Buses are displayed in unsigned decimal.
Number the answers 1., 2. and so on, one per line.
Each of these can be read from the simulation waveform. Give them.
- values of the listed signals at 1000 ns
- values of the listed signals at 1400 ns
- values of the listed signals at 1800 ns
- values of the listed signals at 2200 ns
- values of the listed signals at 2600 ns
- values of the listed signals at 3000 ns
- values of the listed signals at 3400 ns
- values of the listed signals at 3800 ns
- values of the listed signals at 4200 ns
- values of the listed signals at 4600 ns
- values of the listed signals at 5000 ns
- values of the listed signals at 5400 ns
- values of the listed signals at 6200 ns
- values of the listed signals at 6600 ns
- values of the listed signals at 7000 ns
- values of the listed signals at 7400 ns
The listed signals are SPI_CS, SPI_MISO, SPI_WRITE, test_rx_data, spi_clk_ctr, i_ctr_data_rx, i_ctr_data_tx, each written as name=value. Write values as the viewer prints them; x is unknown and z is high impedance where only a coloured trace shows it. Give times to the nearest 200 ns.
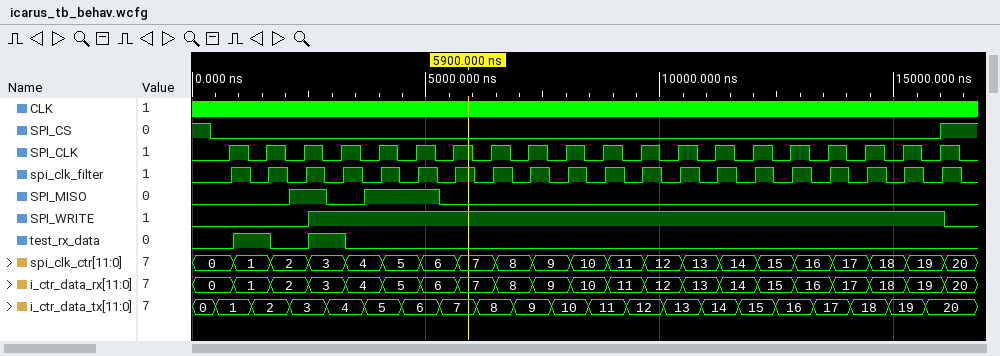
1. SPI_CS=0, SPI_MISO=0, SPI_WRITE=0, test_rx_data=1, spi_clk_ctr=1, i_ctr_data_rx=1, i_ctr_data_tx=1
2. SPI_CS=0, SPI_MISO=0, SPI_WRITE=0, test_rx_data=1, spi_clk_ctr=1, i_ctr_data_rx=1, i_ctr_data_tx=2
3. SPI_CS=0, SPI_MISO=0, SPI_WRITE=0, test_rx_data=0, spi_clk_ctr=2, i_ctr_data_rx=2, i_ctr_data_tx=2
4. SPI_CS=0, SPI_MISO=1, SPI_WRITE=0, test_rx_data=0, spi_clk_ctr=2, i_ctr_data_rx=2, i_ctr_data_tx=3
5. SPI_CS=0, SPI_MISO=1, SPI_WRITE=1, test_rx_data=1, spi_clk_ctr=3, i_ctr_data_rx=3, i_ctr_data_tx=3
6. SPI_CS=0, SPI_MISO=0, SPI_WRITE=1, test_rx_data=1, spi_clk_ctr=3, i_ctr_data_rx=3, i_ctr_data_tx=4
7. SPI_CS=0, SPI_MISO=0, SPI_WRITE=1, test_rx_data=0, spi_clk_ctr=4, i_ctr_data_rx=4, i_ctr_data_tx=4
8. SPI_CS=0, SPI_MISO=1, SPI_WRITE=1, test_rx_data=0, spi_clk_ctr=4, i_ctr_data_rx=4, i_ctr_data_tx=5
9. SPI_CS=0, SPI_MISO=1, SPI_WRITE=1, test_rx_data=0, spi_clk_ctr=5, i_ctr_data_rx=5, i_ctr_data_tx=5
10. SPI_CS=0, SPI_MISO=1, SPI_WRITE=1, test_rx_data=0, spi_clk_ctr=5, i_ctr_data_rx=5, i_ctr_data_tx=6
11. SPI_CS=0, SPI_MISO=1, SPI_WRITE=1, test_rx_data=0, spi_clk_ctr=6, i_ctr_data_rx=6, i_ctr_data_tx=6
12. SPI_CS=0, SPI_MISO=0, SPI_WRITE=1, test_rx_data=0, spi_clk_ctr=6, i_ctr_data_rx=6, i_ctr_data_tx=7
13. SPI_CS=0, SPI_MISO=0, SPI_WRITE=1, test_rx_data=0, spi_clk_ctr=7, i_ctr_data_rx=7, i_ctr_data_tx=8
14. SPI_CS=0, SPI_MISO=0, SPI_WRITE=1, test_rx_data=0, spi_clk_ctr=8, i_ctr_data_rx=8, i_ctr_data_tx=8
15. SPI_CS=0, SPI_MISO=0, SPI_WRITE=1, test_rx_data=0, spi_clk_ctr=8, i_ctr_data_rx=8, i_ctr_data_tx=9
16. SPI_CS=0, SPI_MISO=0, SPI_WRITE=1, test_rx_data=0, spi_clk_ctr=9, i_ctr_data_rx=9, i_ctr_data_tx=9
